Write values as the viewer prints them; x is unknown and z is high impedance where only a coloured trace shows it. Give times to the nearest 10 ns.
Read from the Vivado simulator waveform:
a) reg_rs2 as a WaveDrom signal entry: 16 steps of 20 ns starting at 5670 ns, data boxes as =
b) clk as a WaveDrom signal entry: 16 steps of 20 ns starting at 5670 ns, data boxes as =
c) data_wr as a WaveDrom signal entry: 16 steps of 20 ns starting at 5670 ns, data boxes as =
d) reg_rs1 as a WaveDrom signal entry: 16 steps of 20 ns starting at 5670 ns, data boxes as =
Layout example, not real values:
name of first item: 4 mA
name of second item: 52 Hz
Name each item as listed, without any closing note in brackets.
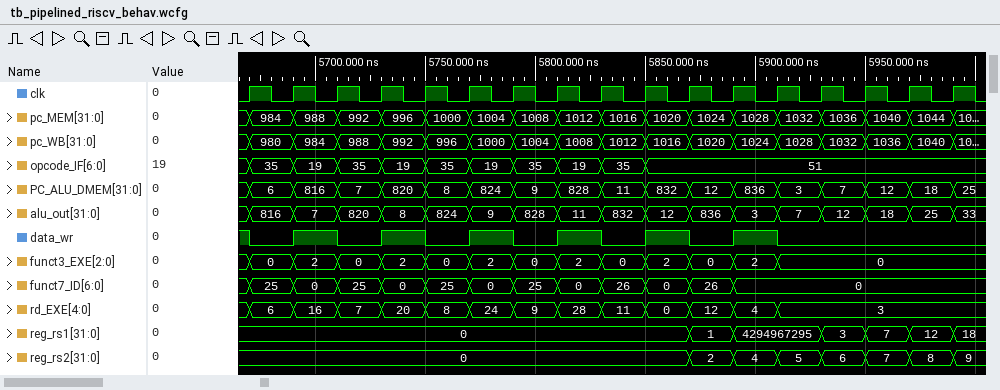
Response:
reg_rs2 as a WaveDrom signal entry: 16 steps of 20 ns starting at 5670 ns, data boxes as =: {name: 'reg_rs2', wave: '=.........======', data: '0 2 4 5 6 7 8'}
clk as a WaveDrom signal entry: 16 steps of 20 ns starting at 5670 ns, data boxes as =: {name: 'clk', wave: 'p...............'}
data_wr as a WaveDrom signal entry: 16 steps of 20 ns starting at 5670 ns, data boxes as =: {name: 'data_wr', wave: '0101010101010...'}
reg_rs1 as a WaveDrom signal entry: 16 steps of 20 ns starting at 5670 ns, data boxes as =: {name: 'reg_rs1', wave: '=.........==.===', data: '0 1 4294967295 3 7 12'}
